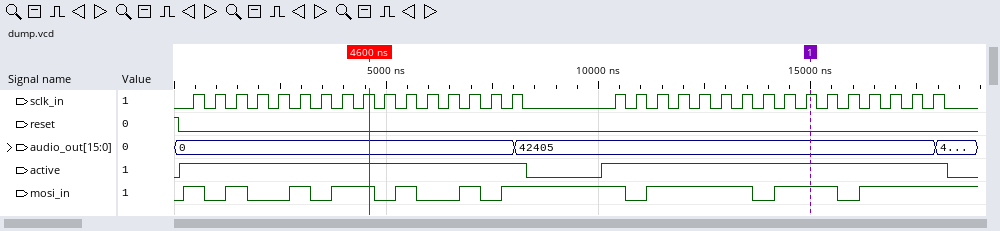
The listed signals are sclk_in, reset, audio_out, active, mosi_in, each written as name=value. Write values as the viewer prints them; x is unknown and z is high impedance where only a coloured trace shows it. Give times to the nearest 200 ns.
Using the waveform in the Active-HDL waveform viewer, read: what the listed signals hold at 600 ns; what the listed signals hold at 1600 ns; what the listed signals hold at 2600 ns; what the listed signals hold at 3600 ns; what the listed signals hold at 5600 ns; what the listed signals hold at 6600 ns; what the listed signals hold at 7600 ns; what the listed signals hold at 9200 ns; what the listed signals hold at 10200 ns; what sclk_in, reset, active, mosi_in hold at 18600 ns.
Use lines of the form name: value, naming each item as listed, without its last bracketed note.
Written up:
what the listed signals hold at 600 ns: sclk_in=1, reset=0, audio_out=0, active=1, mosi_in=1
what the listed signals hold at 1600 ns: sclk_in=1, reset=0, audio_out=0, active=1, mosi_in=1
what the listed signals hold at 2600 ns: sclk_in=1, reset=0, audio_out=0, active=1, mosi_in=0
what the listed signals hold at 3600 ns: sclk_in=1, reset=0, audio_out=0, active=1, mosi_in=0
what the listed signals hold at 5600 ns: sclk_in=1, reset=0, audio_out=0, active=1, mosi_in=1
what the listed signals hold at 6600 ns: sclk_in=1, reset=0, audio_out=0, active=1, mosi_in=0
what the listed signals hold at 7600 ns: sclk_in=1, reset=0, audio_out=0, active=1, mosi_in=0
what the listed signals hold at 9200 ns: sclk_in=0, reset=0, audio_out=42405, active=0, mosi_in=1
what the listed signals hold at 10200 ns: sclk_in=0, reset=0, audio_out=42405, active=1, mosi_in=1
what sclk_in, reset, active, mosi_in hold at 18600 ns: sclk_in=0, reset=0, active=0, mosi_in=1
